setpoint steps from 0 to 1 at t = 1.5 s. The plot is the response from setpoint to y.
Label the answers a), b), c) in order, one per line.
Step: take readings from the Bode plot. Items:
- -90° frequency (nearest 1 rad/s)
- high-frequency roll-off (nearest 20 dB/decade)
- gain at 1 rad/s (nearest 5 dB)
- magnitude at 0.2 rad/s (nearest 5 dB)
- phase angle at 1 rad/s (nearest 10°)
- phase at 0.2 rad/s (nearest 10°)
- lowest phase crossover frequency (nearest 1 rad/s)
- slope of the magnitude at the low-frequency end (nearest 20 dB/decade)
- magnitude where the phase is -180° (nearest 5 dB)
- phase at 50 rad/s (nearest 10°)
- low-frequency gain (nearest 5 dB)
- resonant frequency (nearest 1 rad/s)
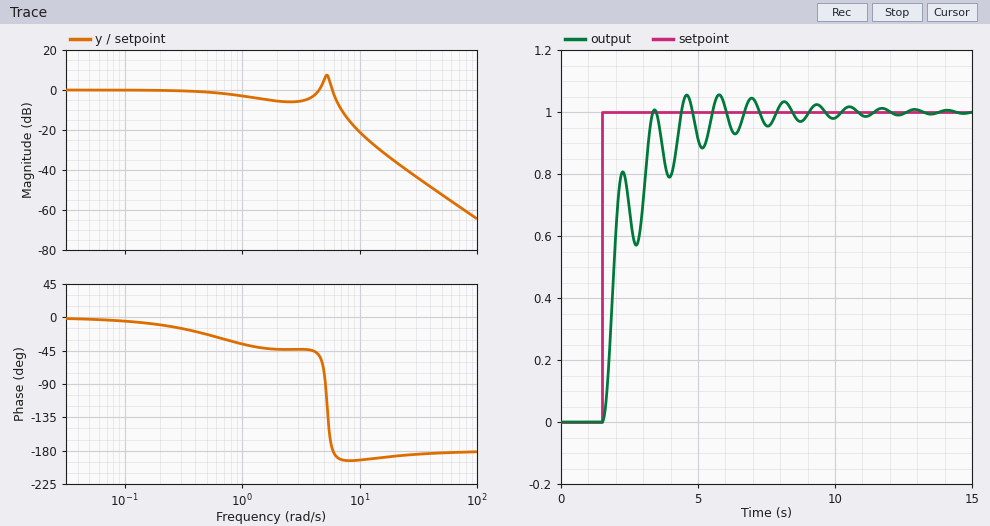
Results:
a) 5 rad/s
b) -40 dB/decade
c) -5 dB
d) 0 dB
e) -40°
f) -10°
g) 6 rad/s
h) 0 dB/decade
i) 0 dB
j) -180°
k) 0 dB
l) 5 rad/s
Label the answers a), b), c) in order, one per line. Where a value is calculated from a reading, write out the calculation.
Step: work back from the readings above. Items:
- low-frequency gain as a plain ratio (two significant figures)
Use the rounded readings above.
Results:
a) 10^(0 / 20) = 1.0
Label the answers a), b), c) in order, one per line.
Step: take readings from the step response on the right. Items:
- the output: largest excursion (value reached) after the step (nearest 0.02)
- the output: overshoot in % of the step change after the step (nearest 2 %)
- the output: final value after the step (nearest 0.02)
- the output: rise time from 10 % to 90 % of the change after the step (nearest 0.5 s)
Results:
a) 1.06
b) 6 %
c) 1.00
d) 1.5 s
